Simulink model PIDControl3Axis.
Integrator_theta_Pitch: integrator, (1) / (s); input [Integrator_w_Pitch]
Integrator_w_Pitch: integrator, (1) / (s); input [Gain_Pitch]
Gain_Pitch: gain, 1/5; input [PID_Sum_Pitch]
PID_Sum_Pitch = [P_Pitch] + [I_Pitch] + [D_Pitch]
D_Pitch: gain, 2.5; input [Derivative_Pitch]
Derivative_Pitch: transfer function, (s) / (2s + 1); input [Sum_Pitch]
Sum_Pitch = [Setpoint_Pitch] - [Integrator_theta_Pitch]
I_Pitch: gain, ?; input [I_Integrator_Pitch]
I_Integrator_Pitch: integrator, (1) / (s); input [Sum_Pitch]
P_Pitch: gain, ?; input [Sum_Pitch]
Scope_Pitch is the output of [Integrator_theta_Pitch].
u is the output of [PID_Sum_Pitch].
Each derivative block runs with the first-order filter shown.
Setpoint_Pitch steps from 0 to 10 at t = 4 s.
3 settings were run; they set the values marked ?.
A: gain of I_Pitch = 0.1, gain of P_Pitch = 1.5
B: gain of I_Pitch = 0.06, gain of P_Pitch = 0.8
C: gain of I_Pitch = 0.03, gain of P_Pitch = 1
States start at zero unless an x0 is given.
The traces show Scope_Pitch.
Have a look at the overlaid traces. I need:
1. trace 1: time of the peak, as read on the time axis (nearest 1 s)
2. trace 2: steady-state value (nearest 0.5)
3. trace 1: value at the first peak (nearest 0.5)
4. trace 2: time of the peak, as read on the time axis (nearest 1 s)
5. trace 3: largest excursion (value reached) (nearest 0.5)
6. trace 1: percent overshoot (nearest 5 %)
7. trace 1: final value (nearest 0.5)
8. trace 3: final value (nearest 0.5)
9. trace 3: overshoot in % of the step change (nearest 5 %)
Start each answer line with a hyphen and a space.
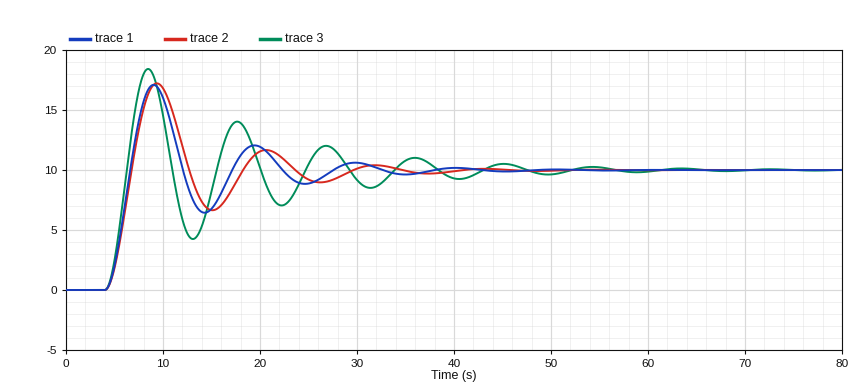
- 9 s
- 10.0
- 17.0
- 9 s
- 18.5
- 70 %
- 10.0
- 10.0
- 85 %
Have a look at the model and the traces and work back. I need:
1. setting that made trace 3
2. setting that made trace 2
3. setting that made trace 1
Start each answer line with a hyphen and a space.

- A
- B
- C
